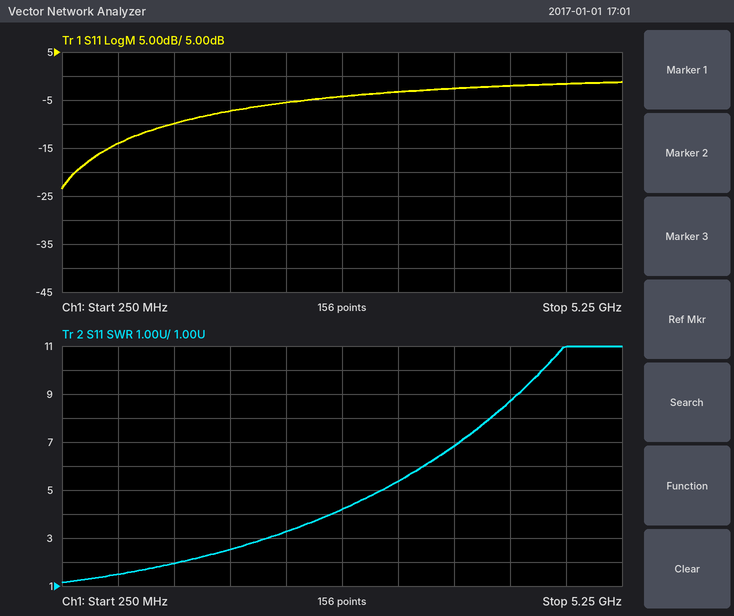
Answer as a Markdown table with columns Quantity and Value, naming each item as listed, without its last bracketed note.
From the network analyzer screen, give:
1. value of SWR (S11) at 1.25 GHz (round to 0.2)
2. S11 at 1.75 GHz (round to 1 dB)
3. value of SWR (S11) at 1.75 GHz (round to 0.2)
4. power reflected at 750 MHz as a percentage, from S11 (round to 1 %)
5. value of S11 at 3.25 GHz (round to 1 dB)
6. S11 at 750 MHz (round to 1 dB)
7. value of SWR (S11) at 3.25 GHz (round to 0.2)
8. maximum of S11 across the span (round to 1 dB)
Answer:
| Quantity | Value |
|---|---|
| value of SWR (S11) at 1.25 GHz | 2.0 |
| S11 at 1.75 GHz | -7 dB |
| value of SWR (S11) at 1.75 GHz | 2.6 |
| power reflected at 750 MHz as a percentage, from S11 | 4 % |
| value of S11 at 3.25 GHz | -3 dB |
| S11 at 750 MHz | -14 dB |
| value of SWR (S11) at 3.25 GHz | 5.4 |
| maximum of S11 across the span | -1 dB |
